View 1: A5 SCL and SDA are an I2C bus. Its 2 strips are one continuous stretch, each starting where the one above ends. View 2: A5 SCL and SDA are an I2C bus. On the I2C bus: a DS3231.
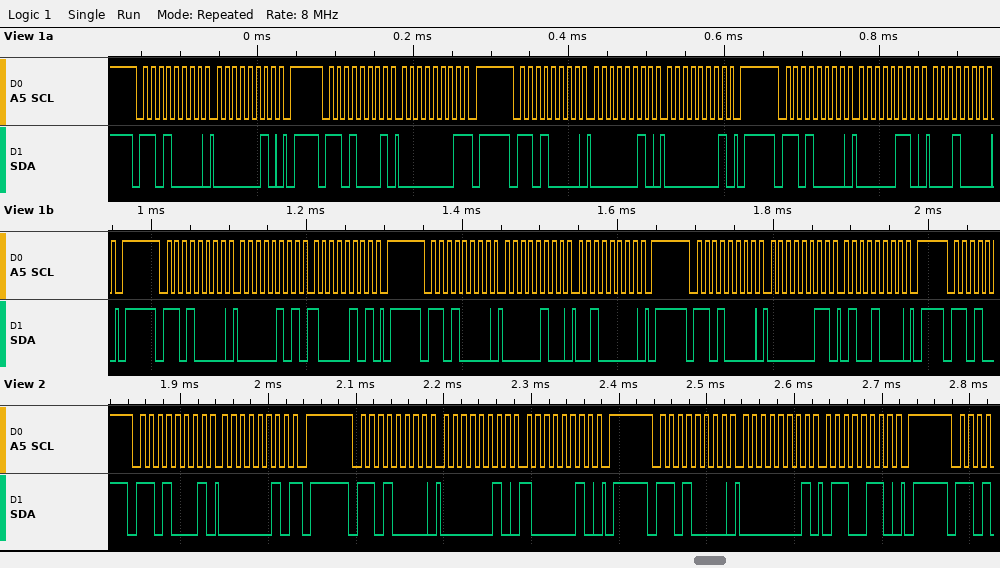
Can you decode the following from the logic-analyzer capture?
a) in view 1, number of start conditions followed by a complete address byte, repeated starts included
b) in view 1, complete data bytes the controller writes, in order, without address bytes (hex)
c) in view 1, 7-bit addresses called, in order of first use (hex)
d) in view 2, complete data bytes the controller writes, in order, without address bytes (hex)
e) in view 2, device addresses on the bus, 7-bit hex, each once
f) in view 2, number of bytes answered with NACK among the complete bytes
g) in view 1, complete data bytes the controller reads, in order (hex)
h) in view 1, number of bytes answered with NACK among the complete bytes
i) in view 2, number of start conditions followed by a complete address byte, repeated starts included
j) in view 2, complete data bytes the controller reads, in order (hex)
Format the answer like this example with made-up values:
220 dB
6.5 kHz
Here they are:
7
02 02 01 06 10 05 85 04 20 03 48
0x68
02 82 01 66
0x68
1
01
1
3
02
